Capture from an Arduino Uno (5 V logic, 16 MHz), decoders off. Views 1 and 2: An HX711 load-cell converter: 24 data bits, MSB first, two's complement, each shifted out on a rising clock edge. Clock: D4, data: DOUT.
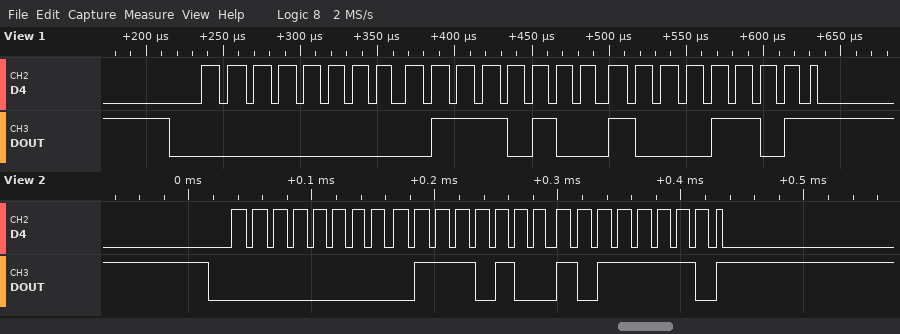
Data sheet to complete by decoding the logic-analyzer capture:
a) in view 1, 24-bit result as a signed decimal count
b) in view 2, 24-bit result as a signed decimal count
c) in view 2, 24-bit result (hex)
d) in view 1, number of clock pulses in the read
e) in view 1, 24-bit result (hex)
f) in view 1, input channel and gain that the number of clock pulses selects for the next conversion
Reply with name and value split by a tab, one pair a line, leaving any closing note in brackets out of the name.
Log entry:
in view 1, 24-bit result as a signed decimal count	29837
in view 2, 24-bit result as a signed decimal count	29886
in view 2, 24-bit result	0x0074BE
in view 1, number of clock pulses in the read	25
in view 1, 24-bit result	0x00748D
in view 1, input channel and gain that the number of clock pulses selects for the next conversion	channel A, gain 128
